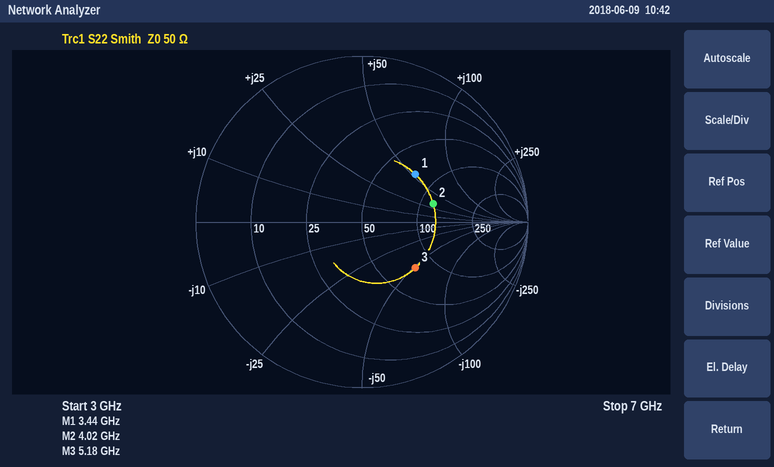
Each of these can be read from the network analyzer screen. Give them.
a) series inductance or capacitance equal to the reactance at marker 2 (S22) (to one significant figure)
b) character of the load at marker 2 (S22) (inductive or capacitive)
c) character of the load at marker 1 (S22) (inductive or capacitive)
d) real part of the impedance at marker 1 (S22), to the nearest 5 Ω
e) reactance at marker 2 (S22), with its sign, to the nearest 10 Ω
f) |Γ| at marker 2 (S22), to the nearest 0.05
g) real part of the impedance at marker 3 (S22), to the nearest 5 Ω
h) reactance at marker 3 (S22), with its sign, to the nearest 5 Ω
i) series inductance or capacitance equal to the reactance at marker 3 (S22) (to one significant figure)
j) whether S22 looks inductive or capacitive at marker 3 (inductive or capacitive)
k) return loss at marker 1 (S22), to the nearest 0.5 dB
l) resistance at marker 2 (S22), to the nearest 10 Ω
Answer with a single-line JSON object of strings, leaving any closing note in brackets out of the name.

{"series inductance or capacitance equal to the reactance at marker 2 (S22)": "1 nH", "character of the load at marker 2 (S22)": "inductive", "character of the load at marker 1 (S22)": "inductive", "real part of the impedance at marker 1 (S22), to the nearest 5 Ω": "75 Ω", "reactance at marker 2 (S22), with its sign, to the nearest 10 Ω": "+30 Ω", "|Γ| at marker 2 (S22), to the nearest 0.05": "0.45", "real part of the impedance at marker 3 (S22), to the nearest 5 Ω": "75 Ω", "reactance at marker 3 (S22), with its sign, to the nearest 5 Ω": "-50 Ω", "series inductance or capacitance equal to the reactance at marker 3 (S22)": "600 fF", "whether S22 looks inductive or capacitive at marker 3": "capacitive", "return loss at marker 1 (S22), to the nearest 0.5 dB": "7.5 dB", "resistance at marker 2 (S22), to the nearest 10 Ω": "120 Ω"}
